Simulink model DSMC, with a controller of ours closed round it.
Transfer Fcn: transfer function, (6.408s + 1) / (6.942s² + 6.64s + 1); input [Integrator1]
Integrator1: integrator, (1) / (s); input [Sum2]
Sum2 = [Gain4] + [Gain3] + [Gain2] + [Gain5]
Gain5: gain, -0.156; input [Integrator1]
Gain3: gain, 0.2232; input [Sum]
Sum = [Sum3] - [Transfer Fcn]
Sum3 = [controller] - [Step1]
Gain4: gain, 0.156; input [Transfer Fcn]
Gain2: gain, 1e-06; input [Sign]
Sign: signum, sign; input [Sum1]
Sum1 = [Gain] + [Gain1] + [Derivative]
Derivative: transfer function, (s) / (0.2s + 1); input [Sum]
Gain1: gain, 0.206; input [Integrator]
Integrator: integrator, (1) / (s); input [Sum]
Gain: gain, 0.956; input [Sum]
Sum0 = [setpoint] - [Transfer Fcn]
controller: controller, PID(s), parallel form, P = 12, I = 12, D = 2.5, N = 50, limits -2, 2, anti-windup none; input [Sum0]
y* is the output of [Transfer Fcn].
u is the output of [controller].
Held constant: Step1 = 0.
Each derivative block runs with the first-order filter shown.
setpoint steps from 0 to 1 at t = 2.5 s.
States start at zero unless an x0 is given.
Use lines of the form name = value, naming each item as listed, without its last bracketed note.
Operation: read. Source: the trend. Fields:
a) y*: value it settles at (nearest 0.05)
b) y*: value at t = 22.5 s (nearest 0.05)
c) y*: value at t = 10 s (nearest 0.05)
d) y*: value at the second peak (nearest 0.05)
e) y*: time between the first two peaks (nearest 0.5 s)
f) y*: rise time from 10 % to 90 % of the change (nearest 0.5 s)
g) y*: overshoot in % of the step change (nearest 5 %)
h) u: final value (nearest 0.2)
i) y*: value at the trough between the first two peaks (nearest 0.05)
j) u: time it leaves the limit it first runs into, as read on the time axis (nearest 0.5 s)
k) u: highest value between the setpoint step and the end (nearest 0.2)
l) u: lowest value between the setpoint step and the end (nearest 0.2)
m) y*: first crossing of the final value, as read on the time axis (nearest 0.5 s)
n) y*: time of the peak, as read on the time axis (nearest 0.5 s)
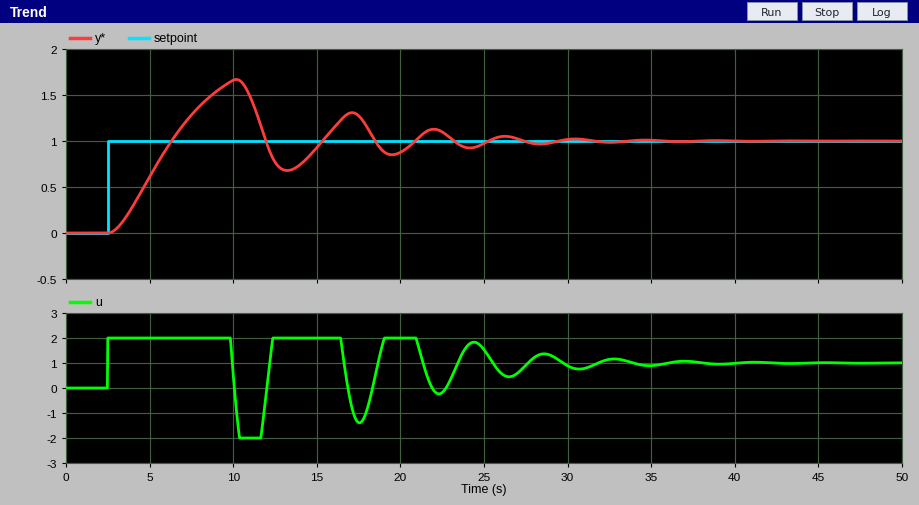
y*: value it settles at = 1.00
y*: value at t = 22.5 s = 1.10
y*: value at t = 10 s = 1.65
y*: value at the second peak = 1.30
y*: time between the first two peaks = 7.0 s
y*: rise time from 10 % to 90 % of the change = 2.5 s
y*: overshoot in % of the step change = 65 %
u: final value = 1.0
y*: value at the trough between the first two peaks = 0.70
u: time it leaves the limit it first runs into, as read on the time axis = 10.0 s
u: highest value between the setpoint step and the end = 2.0
u: lowest value between the setpoint step and the end = -2.0
y*: first crossing of the final value, as read on the time axis = 6.5 s
y*: time of the peak, as read on the time axis = 10.0 s
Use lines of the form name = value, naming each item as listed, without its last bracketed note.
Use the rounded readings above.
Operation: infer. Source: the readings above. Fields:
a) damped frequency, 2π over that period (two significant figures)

damped frequency, 2π over that period = 0.90 rad/s
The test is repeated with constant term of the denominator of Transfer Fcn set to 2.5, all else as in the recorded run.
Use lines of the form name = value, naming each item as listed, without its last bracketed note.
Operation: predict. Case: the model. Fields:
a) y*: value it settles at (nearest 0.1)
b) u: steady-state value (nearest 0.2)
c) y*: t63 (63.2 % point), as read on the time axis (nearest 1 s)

y*: value it settles at = 1.0
u: steady-state value = 2.0
y*: t63 (63.2 % point), as read on the time axis = 5 s
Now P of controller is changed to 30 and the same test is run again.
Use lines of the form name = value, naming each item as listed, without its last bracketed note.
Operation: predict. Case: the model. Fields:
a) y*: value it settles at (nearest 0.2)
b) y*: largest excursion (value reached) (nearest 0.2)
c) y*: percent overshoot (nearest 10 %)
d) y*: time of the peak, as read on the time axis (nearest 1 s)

y*: value it settles at = 1.0
y*: largest excursion (value reached) = 1.6
y*: percent overshoot = 50 %
y*: time of the peak, as read on the time axis = 9 s
